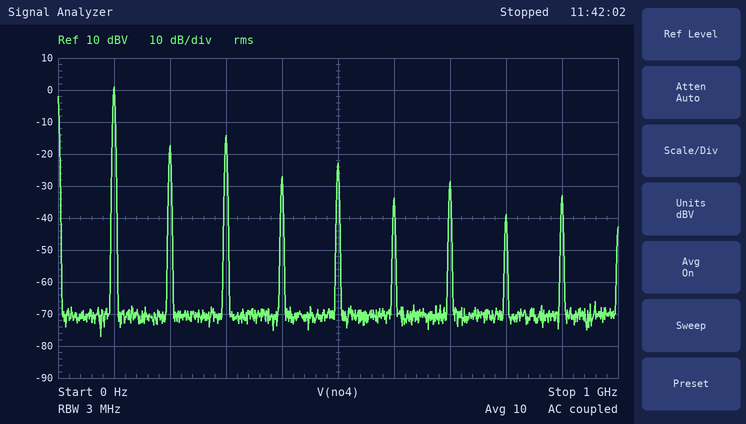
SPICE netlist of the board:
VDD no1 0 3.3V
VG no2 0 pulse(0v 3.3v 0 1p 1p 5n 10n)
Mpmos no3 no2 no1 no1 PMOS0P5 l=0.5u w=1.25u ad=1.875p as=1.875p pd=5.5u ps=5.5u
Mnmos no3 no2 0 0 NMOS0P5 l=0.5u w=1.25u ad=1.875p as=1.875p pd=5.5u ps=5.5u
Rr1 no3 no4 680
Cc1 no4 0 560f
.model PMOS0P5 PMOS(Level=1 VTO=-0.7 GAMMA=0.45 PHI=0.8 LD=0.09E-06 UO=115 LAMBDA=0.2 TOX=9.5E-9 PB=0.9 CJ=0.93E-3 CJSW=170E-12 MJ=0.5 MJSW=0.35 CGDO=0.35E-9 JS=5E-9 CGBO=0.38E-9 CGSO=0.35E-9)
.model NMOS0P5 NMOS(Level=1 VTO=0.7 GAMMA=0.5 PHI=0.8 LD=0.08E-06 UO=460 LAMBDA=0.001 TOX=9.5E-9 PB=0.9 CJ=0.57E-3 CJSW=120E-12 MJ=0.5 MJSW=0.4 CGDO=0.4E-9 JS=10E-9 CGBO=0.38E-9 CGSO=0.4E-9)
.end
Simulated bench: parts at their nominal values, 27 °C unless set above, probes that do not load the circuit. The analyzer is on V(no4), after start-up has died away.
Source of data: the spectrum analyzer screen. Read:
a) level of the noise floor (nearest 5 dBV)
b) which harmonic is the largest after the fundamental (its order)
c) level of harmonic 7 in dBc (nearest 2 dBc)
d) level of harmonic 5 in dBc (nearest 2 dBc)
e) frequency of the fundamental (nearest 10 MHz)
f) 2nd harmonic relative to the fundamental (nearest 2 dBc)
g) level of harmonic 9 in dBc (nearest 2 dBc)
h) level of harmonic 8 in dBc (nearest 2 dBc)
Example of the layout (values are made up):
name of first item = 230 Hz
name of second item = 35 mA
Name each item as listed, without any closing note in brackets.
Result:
level of the noise floor = -70 dBV
which harmonic is the largest after the fundamental = 3
level of harmonic 7 in dBc = -30 dBc
level of harmonic 5 in dBc = -24 dBc
frequency of the fundamental = 100 MHz
2nd harmonic relative to the fundamental = -18 dBc
level of harmonic 9 in dBc = -34 dBc
level of harmonic 8 in dBc = -40 dBc
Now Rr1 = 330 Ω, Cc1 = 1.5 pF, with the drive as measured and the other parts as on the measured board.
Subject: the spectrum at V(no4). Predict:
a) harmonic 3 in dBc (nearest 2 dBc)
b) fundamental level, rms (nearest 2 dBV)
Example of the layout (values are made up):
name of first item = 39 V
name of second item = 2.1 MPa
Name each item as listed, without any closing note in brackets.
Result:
harmonic 3 in dBc = -18 dBc
fundamental level, rms = -4 dBV
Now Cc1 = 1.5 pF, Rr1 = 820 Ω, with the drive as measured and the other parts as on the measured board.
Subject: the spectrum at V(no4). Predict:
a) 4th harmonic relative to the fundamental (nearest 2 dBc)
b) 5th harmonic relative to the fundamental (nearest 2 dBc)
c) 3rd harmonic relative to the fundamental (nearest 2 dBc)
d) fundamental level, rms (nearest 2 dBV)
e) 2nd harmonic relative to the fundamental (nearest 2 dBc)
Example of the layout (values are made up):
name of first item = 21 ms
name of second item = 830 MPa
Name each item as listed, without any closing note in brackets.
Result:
4th harmonic relative to the fundamental = -34 dBc
5th harmonic relative to the fundamental = -28 dBc
3rd harmonic relative to the fundamental = -18 dBc
fundamental level, rms = -4 dBV
2nd harmonic relative to the fundamental = -22 dBc
